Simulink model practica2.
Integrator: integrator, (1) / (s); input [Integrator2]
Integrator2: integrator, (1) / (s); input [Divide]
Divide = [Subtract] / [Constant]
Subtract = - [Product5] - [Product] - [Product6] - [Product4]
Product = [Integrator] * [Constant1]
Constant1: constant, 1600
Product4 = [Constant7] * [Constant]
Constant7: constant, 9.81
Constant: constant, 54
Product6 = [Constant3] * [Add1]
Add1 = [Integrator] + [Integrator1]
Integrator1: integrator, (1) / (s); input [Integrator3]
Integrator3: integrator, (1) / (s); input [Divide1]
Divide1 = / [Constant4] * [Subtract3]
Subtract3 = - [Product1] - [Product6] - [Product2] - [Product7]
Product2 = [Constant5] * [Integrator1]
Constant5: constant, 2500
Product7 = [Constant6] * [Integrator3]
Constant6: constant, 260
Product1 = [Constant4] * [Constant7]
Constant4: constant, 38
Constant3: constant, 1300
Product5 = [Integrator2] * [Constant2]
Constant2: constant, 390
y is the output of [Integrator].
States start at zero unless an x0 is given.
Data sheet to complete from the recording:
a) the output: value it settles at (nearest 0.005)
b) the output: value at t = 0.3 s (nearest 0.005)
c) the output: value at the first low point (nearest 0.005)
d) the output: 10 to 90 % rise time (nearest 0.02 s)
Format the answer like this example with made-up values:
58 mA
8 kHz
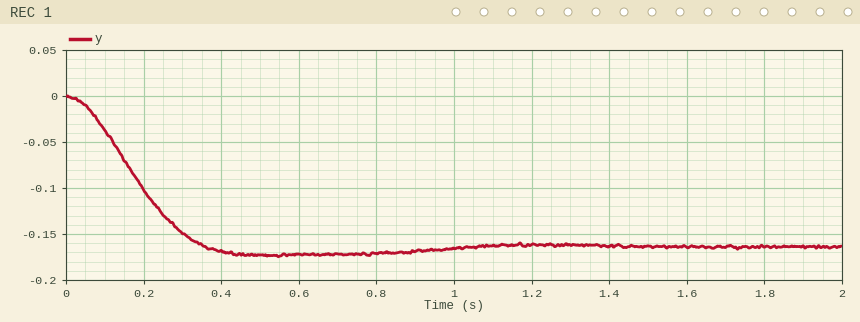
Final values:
-0.165
-0.150
-0.175
0.24 s
